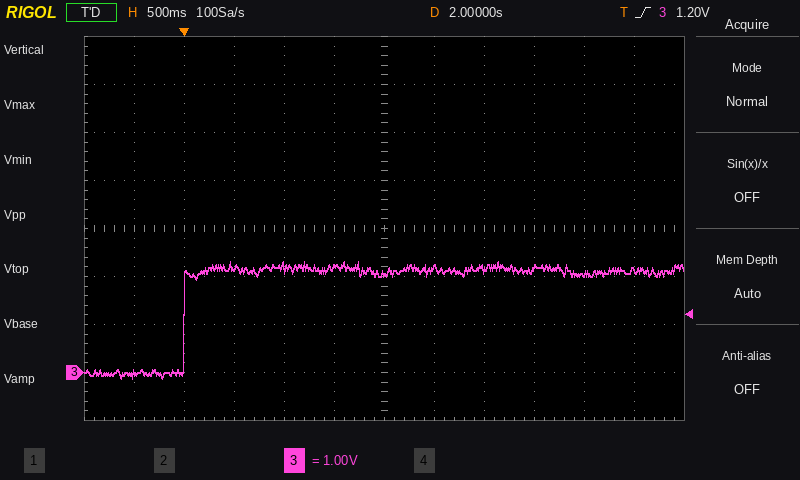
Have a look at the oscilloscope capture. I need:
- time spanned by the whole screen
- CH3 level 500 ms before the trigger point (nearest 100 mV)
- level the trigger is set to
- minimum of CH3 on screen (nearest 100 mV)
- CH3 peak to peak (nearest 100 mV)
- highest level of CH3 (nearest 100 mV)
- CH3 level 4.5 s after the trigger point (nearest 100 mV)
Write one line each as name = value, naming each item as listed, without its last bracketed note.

time spanned by the whole screen = 6 s
CH3 level 500 ms before the trigger point = 0.0 V
level the trigger is set to = 1.20 V
minimum of CH3 on screen = -100 mV
CH3 peak to peak = 2.4 V
highest level of CH3 = 2.3 V
CH3 level 4.5 s after the trigger point = 2.1 V
